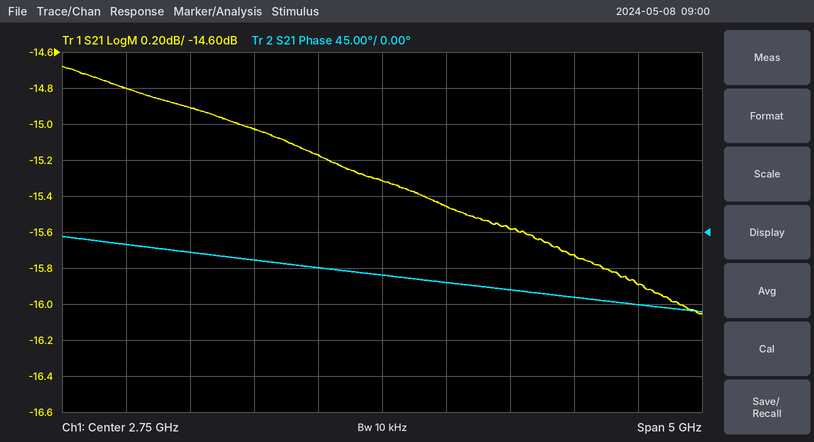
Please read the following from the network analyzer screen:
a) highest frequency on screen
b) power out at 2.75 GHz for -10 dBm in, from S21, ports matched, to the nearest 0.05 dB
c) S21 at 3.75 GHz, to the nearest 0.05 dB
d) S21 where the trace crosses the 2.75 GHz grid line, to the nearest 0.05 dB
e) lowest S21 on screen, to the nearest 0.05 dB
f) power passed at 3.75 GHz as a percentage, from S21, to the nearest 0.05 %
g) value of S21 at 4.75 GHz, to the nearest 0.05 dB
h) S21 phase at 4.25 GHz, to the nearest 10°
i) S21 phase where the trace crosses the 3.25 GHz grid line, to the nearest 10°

5.25 GHz
-25.30 dBm
-15.60 dB
-15.30 dB
-16.05 dB
2.75 %
-15.90 dB
-80°
-60°
